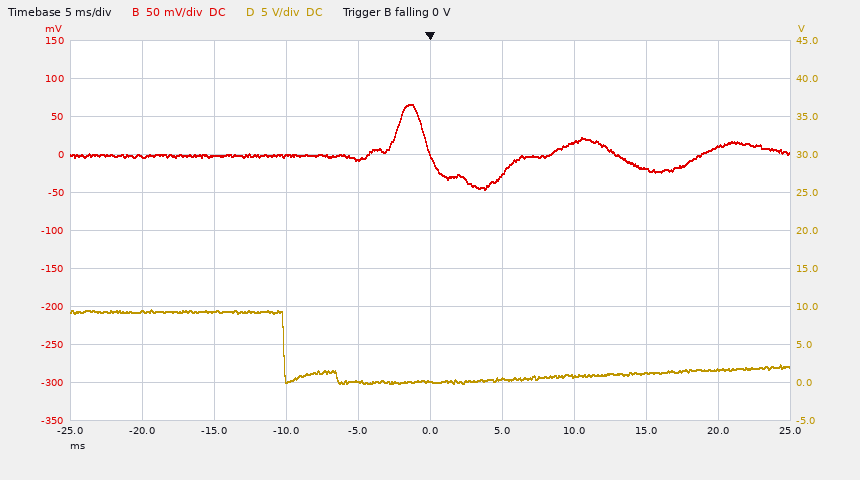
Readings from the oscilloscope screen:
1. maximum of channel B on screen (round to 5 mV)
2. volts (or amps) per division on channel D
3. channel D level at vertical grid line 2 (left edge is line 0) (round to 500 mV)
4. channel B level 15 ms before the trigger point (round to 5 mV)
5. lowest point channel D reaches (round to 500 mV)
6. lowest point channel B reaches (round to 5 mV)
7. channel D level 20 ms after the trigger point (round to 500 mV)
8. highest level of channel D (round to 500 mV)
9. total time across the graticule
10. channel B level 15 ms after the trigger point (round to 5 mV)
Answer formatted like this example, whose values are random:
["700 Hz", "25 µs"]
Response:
["65 mV", "5 V", "9.5 V", "0 mV", "0.0 V", "-45 mV", "1.5 V", "9.5 V", "50 ms", "-20 mV"]
